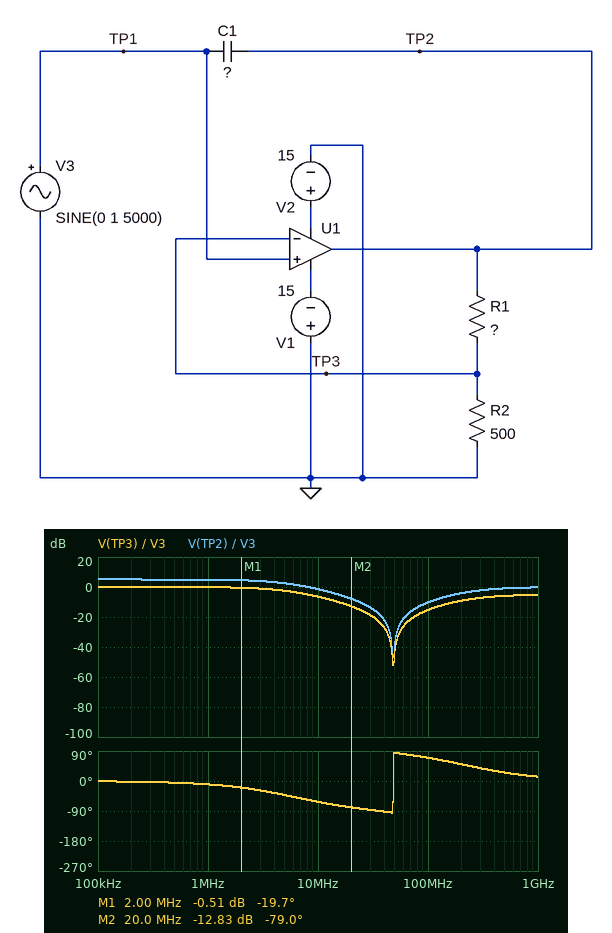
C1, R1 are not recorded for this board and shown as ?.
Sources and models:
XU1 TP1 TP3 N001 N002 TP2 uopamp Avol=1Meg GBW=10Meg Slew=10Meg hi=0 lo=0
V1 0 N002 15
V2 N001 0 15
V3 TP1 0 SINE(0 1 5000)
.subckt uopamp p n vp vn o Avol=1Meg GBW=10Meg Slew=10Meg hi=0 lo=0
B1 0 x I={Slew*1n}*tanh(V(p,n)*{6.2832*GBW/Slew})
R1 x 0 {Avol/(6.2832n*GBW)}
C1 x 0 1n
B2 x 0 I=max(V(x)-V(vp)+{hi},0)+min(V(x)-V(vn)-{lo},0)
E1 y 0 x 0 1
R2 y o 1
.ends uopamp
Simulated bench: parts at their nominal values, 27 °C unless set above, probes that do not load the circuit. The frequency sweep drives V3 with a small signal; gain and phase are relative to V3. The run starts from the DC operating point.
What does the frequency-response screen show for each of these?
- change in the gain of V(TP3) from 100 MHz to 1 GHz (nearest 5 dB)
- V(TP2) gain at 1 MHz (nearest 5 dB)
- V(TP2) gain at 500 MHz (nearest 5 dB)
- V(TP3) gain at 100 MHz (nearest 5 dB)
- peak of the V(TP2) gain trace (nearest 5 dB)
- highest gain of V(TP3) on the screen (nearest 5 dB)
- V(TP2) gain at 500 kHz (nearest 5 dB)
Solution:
10 dB
5 dB
0 dB
-15 dB
5 dB
0 dB
5 dB
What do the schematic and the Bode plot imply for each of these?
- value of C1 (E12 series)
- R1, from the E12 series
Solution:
680 pF
390 Ω
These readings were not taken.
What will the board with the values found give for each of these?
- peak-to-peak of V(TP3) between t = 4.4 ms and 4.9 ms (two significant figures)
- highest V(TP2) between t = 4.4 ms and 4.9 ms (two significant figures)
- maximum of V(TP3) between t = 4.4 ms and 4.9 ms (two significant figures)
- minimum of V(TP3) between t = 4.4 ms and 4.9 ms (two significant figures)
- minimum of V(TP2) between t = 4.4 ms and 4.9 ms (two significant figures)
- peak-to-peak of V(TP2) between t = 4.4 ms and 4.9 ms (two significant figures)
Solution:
2.0 V
1.8 V
1.0 V
-1.0 V
-1.8 V
3.6 V
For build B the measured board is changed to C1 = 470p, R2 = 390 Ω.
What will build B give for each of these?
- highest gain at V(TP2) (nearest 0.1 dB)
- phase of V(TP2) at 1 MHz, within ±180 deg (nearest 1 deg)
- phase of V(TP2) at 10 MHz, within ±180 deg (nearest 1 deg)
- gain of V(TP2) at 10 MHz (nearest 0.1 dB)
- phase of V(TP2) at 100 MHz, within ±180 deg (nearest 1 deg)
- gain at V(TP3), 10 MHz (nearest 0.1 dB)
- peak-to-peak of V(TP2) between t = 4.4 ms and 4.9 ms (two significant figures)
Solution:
6.0 dB
-11 deg
-65 deg
-1.1 dB
76 deg
-7.2 dB
4.0 V
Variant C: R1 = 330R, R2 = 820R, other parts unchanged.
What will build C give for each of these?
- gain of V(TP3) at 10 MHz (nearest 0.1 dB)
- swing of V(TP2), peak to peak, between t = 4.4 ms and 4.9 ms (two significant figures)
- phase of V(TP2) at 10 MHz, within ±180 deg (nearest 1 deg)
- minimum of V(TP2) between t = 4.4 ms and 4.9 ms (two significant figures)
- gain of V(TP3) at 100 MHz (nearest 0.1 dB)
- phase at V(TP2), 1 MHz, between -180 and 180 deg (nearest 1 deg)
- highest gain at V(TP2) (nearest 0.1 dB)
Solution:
-4.9 dB
2.8 V
-56 deg
-1.4 V
-13.2 dB
-8 deg
2.9 dB
